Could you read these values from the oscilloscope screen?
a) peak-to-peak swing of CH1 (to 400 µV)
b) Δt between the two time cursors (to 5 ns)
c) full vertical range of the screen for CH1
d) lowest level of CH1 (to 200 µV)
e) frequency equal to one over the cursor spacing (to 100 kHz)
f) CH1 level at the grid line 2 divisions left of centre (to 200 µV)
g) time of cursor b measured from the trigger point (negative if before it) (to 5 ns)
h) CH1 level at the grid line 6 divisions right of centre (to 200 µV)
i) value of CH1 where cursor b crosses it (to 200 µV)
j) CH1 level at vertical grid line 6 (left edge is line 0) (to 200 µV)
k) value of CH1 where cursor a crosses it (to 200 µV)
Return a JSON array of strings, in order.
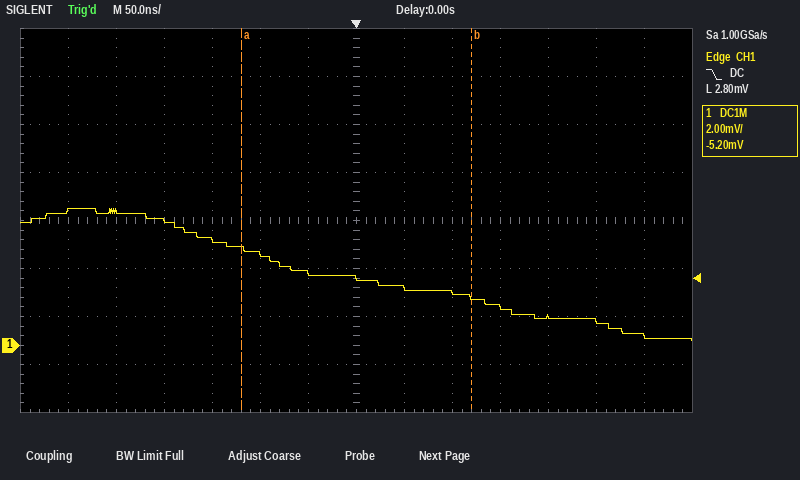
["5.6 mV", "240 ns", "16 mV", "200 µV", "4.2 MHz", "3.8 mV", "+120 ns", "400 µV", "2.0 mV", "3.0 mV", "4.0 mV"]
